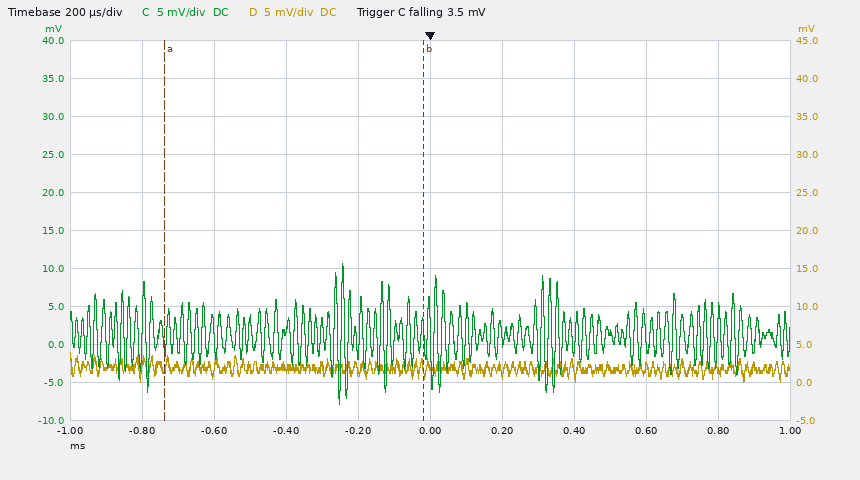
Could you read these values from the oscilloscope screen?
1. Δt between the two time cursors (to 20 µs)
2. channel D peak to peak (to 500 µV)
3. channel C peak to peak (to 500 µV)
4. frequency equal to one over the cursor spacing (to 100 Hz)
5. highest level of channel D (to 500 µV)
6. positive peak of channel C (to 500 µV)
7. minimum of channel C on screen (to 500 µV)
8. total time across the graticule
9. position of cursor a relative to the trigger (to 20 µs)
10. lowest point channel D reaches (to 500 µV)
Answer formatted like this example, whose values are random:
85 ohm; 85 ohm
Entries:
720 µs; 4.0 mV; 18.5 mV; 1.4 kHz; 4.0 mV; 10.5 mV; -8.0 mV; 2 ms; -740 µs; 0.0 mV
